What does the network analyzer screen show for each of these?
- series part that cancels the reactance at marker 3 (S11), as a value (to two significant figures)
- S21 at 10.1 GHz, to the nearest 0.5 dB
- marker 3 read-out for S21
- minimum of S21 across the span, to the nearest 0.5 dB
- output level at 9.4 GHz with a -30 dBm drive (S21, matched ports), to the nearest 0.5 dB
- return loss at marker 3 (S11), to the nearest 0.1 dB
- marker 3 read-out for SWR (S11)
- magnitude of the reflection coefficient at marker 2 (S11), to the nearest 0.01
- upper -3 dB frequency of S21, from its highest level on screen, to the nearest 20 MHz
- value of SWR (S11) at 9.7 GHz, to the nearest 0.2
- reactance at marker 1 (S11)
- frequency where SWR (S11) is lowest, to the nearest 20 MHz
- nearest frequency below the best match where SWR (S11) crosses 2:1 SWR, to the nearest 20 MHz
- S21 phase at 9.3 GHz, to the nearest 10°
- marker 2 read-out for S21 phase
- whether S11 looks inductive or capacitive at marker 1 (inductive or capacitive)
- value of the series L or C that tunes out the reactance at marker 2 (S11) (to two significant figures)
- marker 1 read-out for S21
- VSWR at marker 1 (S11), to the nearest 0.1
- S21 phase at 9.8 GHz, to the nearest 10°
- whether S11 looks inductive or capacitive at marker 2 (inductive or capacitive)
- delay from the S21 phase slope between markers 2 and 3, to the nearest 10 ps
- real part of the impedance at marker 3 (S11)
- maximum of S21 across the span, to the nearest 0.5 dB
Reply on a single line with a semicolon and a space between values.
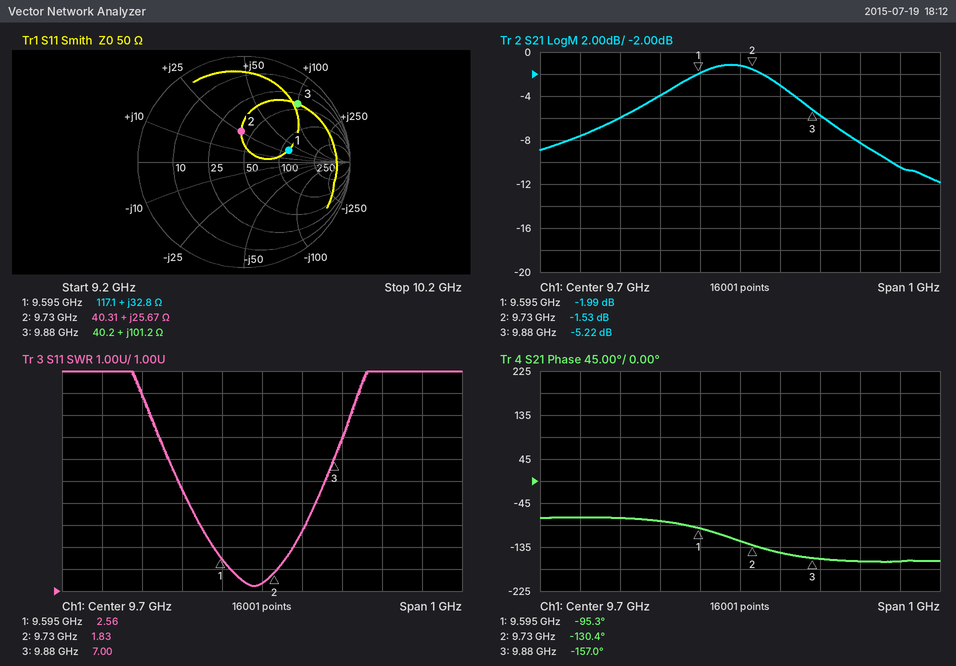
160 fF; -10.5 dB; -5.22 dB; -12.0 dB; -36.0 dBm; 2.5 dB; 7.00; 0.29; 9.84 GHz; 1.4; +32.8 Ω; 9.68 GHz; 9.62 GHz; -70°; -130.4°; inductive; 640 fF; -1.99 dB; 2.6; -150°; inductive; 490 ps; 40.2 Ω; -1.0 dB
